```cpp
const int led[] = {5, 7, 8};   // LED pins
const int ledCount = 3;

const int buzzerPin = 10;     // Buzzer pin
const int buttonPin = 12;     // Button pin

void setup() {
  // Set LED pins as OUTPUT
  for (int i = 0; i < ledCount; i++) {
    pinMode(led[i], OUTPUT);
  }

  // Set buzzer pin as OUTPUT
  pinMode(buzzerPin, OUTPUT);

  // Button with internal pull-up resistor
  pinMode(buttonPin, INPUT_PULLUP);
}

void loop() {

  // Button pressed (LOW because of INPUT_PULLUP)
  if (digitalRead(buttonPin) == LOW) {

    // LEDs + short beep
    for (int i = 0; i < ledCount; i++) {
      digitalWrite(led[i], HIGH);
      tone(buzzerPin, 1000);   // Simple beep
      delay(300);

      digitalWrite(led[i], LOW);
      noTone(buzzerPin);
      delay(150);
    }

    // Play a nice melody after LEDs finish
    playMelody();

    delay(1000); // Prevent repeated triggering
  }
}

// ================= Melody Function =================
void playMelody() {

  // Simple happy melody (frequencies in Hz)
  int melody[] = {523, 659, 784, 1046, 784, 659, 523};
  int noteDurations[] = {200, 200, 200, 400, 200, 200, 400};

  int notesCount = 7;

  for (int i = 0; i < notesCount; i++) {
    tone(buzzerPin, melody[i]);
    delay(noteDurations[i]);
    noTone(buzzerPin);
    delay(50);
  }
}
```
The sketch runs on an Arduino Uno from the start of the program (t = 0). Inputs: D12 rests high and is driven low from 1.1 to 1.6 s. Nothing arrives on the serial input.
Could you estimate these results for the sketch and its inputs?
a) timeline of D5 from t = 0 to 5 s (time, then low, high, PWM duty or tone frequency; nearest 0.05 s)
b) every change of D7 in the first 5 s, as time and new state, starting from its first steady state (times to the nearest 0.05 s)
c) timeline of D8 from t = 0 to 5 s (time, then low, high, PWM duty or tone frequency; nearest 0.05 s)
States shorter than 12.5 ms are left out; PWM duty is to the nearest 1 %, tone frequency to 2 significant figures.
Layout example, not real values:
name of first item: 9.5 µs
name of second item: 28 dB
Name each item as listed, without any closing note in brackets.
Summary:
timeline of D5 from t = 0 to 5 s: 0 s low; 1.1 s high; 1.4 s low
every change of D7 in the first 5 s, as time and new state, starting from its first steady state: 0 s low; 1.55 s high; 1.85 s low
timeline of D8 from t = 0 to 5 s: 0 s low; 2 s high; 2.3 s low
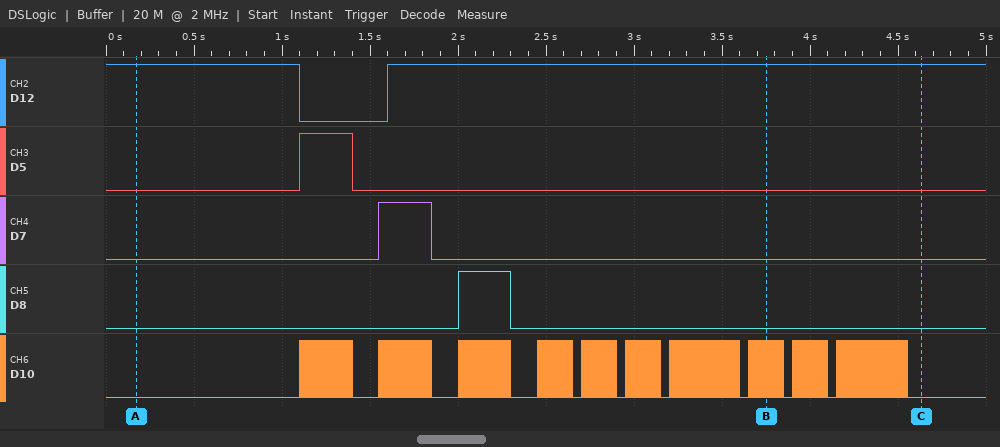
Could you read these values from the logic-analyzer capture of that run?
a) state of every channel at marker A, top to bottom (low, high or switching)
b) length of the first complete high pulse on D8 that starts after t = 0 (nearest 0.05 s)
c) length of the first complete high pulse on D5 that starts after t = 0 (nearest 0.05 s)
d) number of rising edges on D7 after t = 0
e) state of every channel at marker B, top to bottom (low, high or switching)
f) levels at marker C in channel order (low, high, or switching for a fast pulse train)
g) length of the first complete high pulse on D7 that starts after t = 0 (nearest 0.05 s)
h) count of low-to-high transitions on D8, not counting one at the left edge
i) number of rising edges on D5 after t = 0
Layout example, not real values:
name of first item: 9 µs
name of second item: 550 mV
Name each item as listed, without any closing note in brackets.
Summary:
state of every channel at marker A, top to bottom: D12 high, D5 low, D7 low, D8 low, D10 low
length of the first complete high pulse on D8 that starts after t = 0: 0.30 s
length of the first complete high pulse on D5 that starts after t = 0: 0.30 s
number of rising edges on D7 after t = 0: 1
state of every channel at marker B, top to bottom: D12 high, D5 low, D7 low, D8 low, D10 switching
levels at marker C in channel order: D12 high, D5 low, D7 low, D8 low, D10 low
length of the first complete high pulse on D7 that starts after t = 0: 0.30 s
count of low-to-high transitions on D8, not counting one at the left edge: 1
number of rising edges on D5 after t = 0: 1
